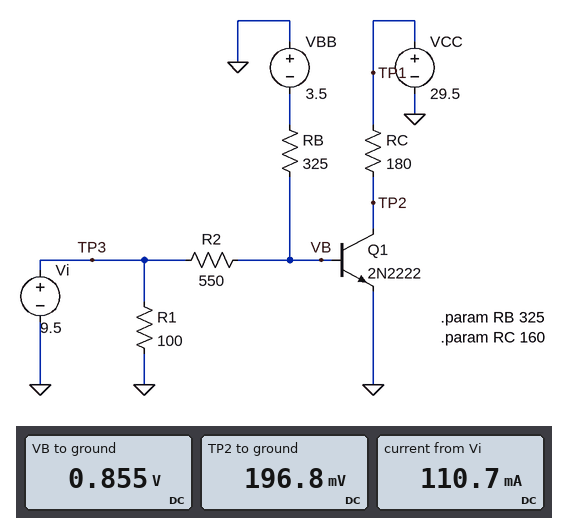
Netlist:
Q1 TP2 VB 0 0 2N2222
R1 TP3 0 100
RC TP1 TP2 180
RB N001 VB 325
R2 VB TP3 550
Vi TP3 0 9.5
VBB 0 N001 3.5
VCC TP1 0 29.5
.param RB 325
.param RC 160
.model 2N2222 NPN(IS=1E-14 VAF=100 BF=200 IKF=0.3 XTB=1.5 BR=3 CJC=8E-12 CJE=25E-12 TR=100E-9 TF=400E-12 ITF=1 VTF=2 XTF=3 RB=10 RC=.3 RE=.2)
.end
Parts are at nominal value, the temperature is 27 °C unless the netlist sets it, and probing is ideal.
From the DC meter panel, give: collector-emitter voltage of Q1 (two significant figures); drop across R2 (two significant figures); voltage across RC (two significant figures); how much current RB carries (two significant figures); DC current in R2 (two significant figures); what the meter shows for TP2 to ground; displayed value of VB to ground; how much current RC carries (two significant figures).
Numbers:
200 mV
8.6 V
29 V
13 mA
16 mA
196.8 mV
0.855 V
160 mA
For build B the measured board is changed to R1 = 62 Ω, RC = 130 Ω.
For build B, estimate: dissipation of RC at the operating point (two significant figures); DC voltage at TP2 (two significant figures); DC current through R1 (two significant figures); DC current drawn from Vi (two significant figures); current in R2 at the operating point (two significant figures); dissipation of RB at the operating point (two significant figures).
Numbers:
6.6 W
280 mV
150 mA
170 mA
16 mA
59 mW
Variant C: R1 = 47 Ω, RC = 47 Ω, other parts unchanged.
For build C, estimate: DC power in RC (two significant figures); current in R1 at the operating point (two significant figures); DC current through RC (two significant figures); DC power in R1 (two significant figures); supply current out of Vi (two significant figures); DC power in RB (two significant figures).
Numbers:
3.6 W
200 mA
280 mA
1.9 W
220 mA
59 mW
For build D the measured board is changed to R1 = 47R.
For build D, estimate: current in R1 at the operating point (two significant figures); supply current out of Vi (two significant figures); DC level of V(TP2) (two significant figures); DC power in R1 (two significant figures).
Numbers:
200 mA
220 mA
200 mV
1.9 W
